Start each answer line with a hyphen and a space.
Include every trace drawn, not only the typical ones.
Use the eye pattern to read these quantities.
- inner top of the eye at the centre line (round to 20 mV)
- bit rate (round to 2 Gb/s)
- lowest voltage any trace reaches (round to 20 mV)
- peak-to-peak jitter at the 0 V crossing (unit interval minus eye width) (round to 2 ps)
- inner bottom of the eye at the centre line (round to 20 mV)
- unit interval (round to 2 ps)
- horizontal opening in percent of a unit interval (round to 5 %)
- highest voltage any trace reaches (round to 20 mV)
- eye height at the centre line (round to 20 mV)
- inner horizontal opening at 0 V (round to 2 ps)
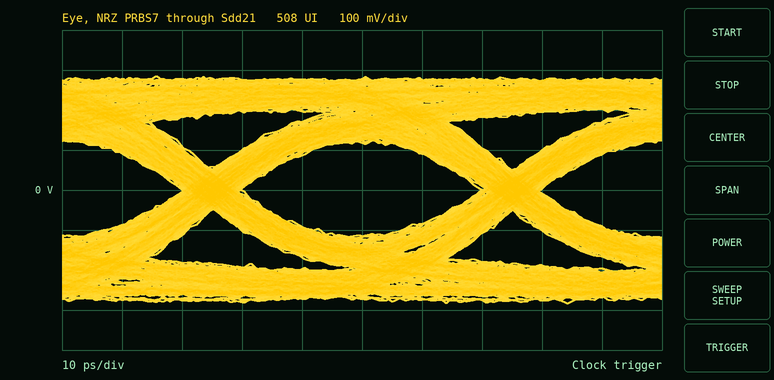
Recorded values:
- 120 mV
- 20 Gb/s
- -280 mV
- 10 ps
- -120 mV
- 50 ps
- 80 %
- 280 mV
- 240 mV
- 40 ps
